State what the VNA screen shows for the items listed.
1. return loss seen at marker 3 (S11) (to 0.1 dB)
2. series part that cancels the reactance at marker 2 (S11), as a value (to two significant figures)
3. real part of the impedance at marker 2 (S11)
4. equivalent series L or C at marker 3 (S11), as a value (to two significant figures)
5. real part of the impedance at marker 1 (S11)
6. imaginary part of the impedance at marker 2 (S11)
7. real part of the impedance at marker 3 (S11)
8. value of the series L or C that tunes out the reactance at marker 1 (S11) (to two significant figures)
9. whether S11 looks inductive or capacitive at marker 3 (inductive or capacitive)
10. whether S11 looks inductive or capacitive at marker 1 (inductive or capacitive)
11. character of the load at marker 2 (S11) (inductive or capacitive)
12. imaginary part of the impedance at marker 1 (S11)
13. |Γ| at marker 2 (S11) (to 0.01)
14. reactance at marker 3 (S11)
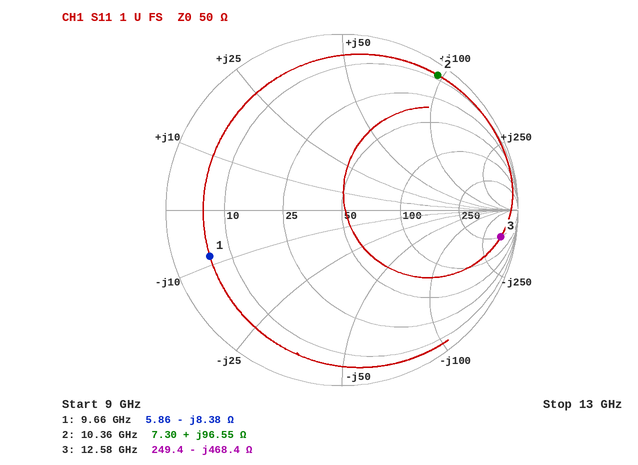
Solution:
0.8 dB
160 fF
7.30 Ω
27 fF
5.86 Ω
+96.55 Ω
249.4 Ω
140 pH
capacitive
capacitive
inductive
-8.38 Ω
0.94
-468.4 Ω
